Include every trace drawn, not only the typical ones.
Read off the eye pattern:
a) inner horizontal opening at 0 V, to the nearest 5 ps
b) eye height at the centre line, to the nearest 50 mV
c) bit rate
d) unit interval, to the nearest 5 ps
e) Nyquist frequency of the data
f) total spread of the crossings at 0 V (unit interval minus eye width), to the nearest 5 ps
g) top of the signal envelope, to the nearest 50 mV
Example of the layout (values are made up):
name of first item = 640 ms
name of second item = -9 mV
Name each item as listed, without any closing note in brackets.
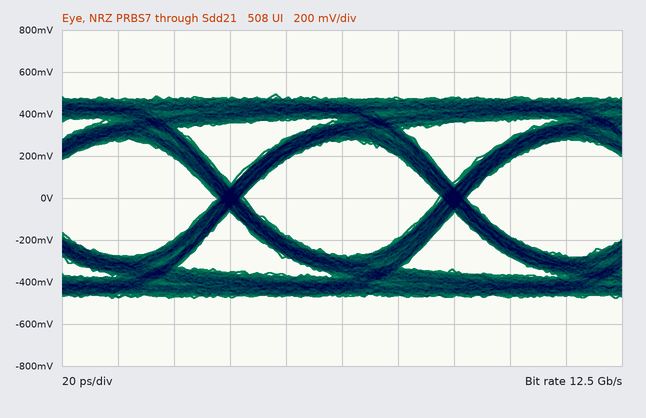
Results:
inner horizontal opening at 0 V, to the nearest 5 ps = 70 ps
eye height at the centre line, to the nearest 50 mV = 550 mV
bit rate = 12.5 Gb/s
unit interval, to the nearest 5 ps = 80 ps
Nyquist frequency of the data = 6.25 GHz
total spread of the crossings at 0 V (unit interval minus eye width), to the nearest 5 ps = 10 ps
top of the signal envelope, to the nearest 50 mV = 500 mV
